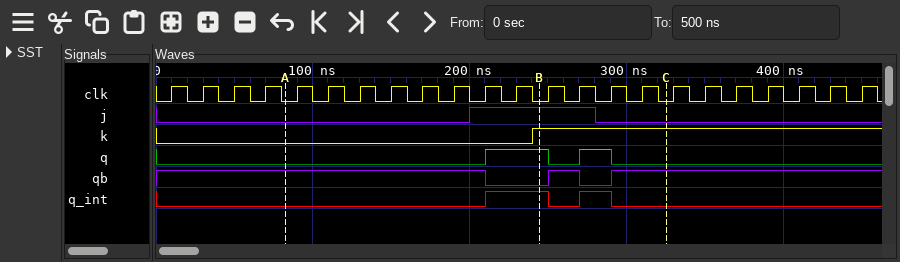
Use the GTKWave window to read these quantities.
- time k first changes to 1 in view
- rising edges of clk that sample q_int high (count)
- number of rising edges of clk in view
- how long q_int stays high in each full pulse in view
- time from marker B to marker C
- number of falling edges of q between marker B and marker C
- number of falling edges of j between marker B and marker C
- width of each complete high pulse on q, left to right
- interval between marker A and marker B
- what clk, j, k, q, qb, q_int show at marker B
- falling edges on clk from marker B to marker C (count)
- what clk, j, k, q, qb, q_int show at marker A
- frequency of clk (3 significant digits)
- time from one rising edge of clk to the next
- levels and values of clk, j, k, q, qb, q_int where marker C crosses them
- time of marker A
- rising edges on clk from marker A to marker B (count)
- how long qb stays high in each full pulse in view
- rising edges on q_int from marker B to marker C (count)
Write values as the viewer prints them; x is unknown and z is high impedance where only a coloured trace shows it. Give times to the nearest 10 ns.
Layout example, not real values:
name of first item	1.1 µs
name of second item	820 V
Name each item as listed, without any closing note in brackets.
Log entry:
time k first changes to 1 in view	240 ns
rising edges of clk that sample q_int high	3
number of rising edges of clk in view	23
how long q_int stays high in each full pulse in view	40 ns, 20 ns
time from marker B to marker C	80 ns
number of falling edges of q between marker B and marker C	2
number of falling edges of j between marker B and marker C	1
width of each complete high pulse on q, left to right	40 ns, 20 ns
interval between marker A and marker B	160 ns
what clk, j, k, q, qb, q_int show at marker B	clk=0, j=1, k=1, q=1, qb=0, q_int=1
falling edges on clk from marker B to marker C	4
what clk, j, k, q, qb, q_int show at marker A	clk=0, j=0, k=0, q=0, qb=1, q_int=0
frequency of clk	50.0 MHz
time from one rising edge of clk to the next	20 ns
levels and values of clk, j, k, q, qb, q_int where marker C crosses them	clk=0, j=0, k=1, q=0, qb=1, q_int=0
time of marker A	80 ns
rising edges on clk from marker A to marker B	8
how long qb stays high in each full pulse in view	20 ns
rising edges on q_int from marker B to marker C	1
